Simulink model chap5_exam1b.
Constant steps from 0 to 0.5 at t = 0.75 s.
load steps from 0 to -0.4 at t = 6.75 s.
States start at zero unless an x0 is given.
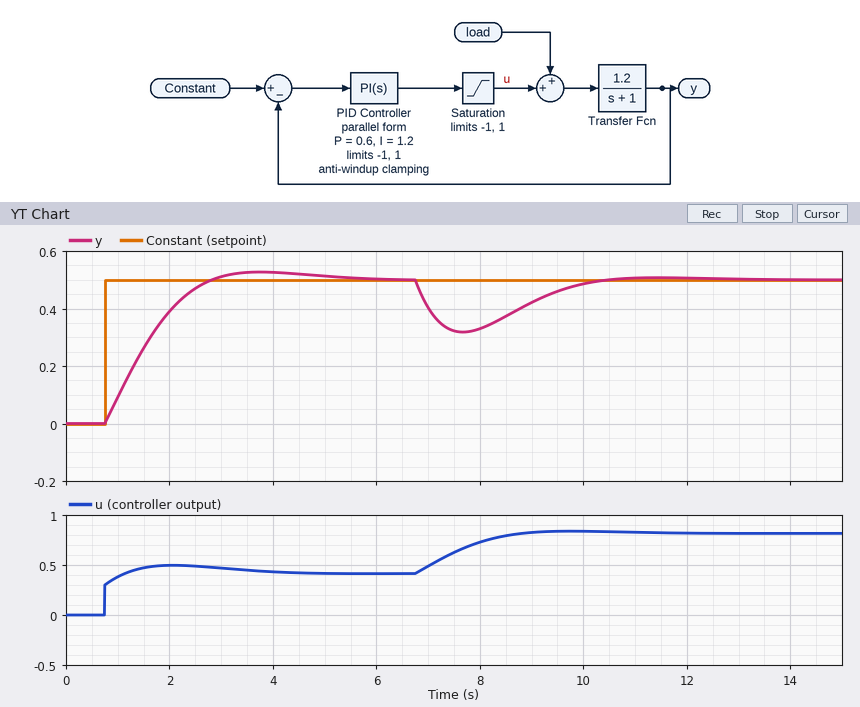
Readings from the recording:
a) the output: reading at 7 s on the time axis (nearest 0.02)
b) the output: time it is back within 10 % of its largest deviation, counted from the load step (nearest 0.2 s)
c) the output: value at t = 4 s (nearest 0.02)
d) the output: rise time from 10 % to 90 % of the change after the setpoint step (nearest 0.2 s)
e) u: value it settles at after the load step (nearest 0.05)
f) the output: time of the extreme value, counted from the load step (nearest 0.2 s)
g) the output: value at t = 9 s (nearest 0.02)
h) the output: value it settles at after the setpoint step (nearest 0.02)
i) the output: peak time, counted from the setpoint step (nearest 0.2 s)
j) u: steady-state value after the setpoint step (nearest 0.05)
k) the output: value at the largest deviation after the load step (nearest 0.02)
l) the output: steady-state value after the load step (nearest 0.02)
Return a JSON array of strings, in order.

["0.40", "3.2 s", "0.52", "1.4 s", "0.80", "1.0 s", "0.42", "0.50", "3.0 s", "0.40", "0.32", "0.50"]
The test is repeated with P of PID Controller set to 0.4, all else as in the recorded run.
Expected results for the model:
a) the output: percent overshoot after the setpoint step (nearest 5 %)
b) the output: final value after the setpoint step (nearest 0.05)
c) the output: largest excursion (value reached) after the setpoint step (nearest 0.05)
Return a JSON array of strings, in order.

["10 %", "0.50", "0.55"]
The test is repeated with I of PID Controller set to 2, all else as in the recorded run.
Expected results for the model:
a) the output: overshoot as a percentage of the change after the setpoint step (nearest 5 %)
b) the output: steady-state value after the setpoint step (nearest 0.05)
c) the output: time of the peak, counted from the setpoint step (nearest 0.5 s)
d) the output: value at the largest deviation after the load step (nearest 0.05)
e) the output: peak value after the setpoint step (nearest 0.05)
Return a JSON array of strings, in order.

["15 %", "0.50", "2.0 s", "0.35", "0.55"]
